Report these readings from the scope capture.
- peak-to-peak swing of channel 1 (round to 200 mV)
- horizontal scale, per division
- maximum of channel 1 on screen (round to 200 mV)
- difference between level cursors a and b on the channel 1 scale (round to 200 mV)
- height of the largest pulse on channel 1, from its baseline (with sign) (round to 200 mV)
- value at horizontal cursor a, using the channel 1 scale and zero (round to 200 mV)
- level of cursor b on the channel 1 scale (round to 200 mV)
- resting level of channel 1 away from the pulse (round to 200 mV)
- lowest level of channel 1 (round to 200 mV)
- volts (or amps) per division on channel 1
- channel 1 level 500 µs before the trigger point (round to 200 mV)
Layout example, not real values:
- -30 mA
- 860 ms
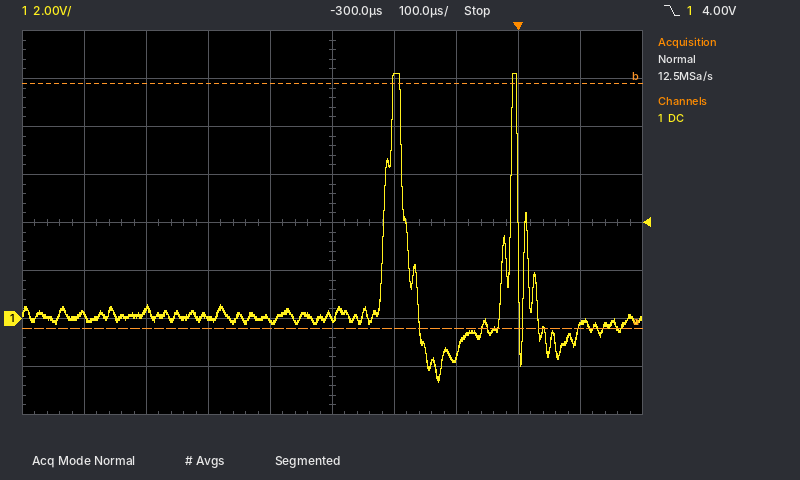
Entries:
- 12.8 V
- 100 µs
- 10.2 V
- 10.2 V
- +10.2 V
- -400 mV
- 9.8 V
- 0.0 V
- -2.6 V
- 2 V
- 0.0 V
